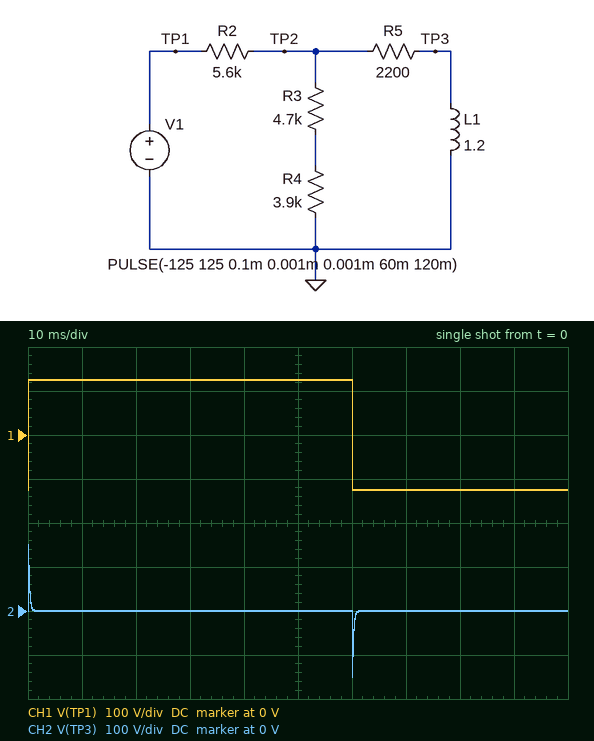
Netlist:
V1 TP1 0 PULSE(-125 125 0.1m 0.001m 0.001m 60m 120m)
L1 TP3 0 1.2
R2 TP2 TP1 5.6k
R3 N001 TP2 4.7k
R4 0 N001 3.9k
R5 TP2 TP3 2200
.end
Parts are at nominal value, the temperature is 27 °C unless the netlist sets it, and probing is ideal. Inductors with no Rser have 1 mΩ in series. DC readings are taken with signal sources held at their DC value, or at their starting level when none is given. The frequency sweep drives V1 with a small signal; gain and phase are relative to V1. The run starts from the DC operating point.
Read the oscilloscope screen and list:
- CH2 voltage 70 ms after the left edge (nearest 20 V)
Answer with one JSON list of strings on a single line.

["0 V"]
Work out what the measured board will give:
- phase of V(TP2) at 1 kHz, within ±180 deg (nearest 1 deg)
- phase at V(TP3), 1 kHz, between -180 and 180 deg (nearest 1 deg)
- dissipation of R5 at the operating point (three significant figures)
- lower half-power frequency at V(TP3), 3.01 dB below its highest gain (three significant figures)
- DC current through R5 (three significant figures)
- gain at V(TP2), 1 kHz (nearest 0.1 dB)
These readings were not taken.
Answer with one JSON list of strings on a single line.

["20 deg", "37 deg", "403 mW", "742 Hz", "13.5 mA", "-5.9 dB"]
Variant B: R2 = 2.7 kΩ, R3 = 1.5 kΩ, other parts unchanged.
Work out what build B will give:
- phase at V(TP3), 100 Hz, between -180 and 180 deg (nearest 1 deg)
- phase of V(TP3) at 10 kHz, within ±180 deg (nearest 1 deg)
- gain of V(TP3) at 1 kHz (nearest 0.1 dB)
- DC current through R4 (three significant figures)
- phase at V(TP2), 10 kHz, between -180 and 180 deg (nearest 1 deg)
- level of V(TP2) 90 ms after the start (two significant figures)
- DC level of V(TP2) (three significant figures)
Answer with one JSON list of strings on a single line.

["79 deg", "3 deg", "-4.6 dB", "8.49 mA", "1 deg", "-46 V", "-45.8 V"]
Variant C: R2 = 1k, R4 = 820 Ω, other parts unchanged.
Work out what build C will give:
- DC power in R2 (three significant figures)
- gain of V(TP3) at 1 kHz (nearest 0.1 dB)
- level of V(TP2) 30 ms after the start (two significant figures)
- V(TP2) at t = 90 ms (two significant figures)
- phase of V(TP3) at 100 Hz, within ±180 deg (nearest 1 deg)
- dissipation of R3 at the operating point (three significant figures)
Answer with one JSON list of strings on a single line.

["2.36 W", "-2.1 dB", "76 V", "-76 V", "76 deg", "901 mW"]
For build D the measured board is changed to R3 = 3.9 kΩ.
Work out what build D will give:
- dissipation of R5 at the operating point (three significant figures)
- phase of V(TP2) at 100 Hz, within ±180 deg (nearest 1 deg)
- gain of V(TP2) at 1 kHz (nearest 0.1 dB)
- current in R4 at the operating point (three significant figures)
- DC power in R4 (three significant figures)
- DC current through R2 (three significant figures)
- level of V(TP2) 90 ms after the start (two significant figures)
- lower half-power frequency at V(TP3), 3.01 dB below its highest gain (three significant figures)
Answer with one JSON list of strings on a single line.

["391 mW", "11 deg", "-6.2 dB", "3.76 mA", "55.1 mW", "17.1 mA", "-29 V", "724 Hz"]
